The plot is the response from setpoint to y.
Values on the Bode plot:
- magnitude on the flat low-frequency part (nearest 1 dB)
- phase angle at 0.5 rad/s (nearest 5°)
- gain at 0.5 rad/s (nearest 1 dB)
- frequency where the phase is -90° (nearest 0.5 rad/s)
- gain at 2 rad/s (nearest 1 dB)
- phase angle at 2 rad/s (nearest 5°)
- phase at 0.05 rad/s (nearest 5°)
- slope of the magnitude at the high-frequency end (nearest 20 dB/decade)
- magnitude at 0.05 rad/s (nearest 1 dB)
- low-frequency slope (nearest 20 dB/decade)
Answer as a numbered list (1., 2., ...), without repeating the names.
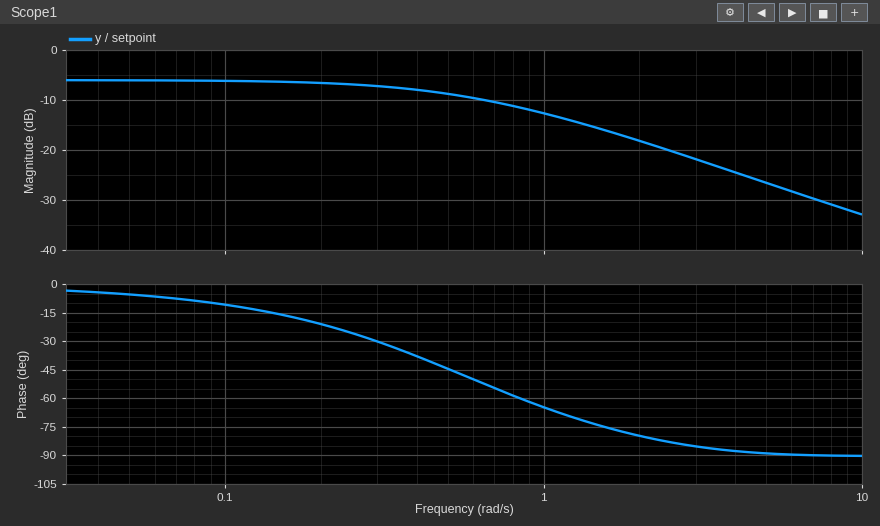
1. -6 dB
2. -45°
3. -9 dB
4. 7.5 rad/s
5. -18 dB
6. -80°
7. -5°
8. -20 dB/decade
9. -6 dB
10. 0 dB/decade
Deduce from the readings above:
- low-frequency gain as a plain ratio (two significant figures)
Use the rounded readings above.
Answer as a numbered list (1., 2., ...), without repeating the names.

1. 0.50
